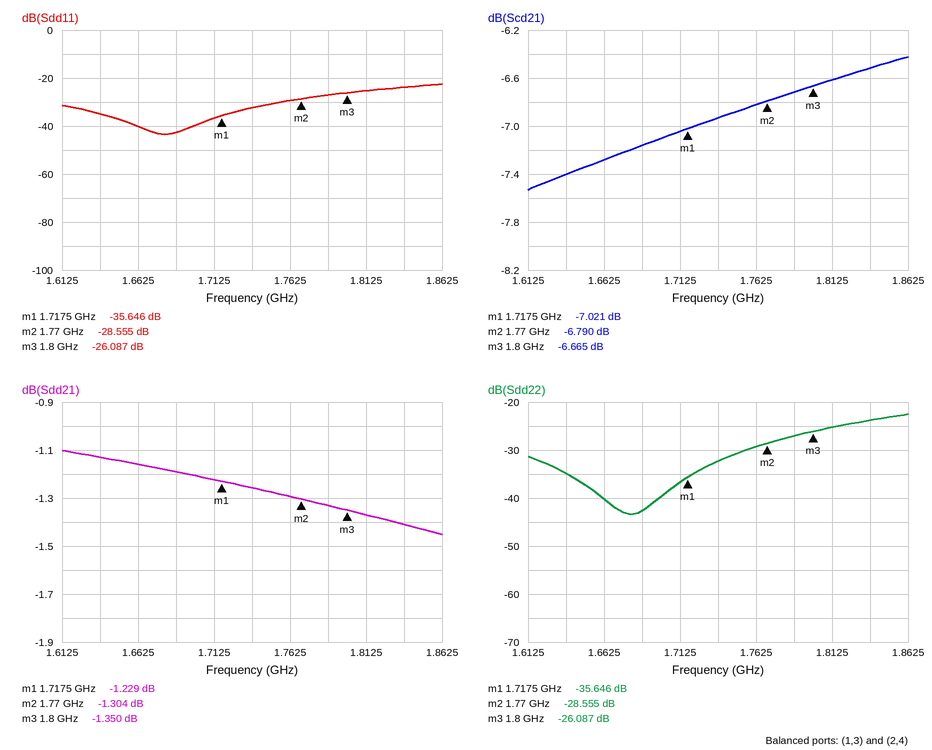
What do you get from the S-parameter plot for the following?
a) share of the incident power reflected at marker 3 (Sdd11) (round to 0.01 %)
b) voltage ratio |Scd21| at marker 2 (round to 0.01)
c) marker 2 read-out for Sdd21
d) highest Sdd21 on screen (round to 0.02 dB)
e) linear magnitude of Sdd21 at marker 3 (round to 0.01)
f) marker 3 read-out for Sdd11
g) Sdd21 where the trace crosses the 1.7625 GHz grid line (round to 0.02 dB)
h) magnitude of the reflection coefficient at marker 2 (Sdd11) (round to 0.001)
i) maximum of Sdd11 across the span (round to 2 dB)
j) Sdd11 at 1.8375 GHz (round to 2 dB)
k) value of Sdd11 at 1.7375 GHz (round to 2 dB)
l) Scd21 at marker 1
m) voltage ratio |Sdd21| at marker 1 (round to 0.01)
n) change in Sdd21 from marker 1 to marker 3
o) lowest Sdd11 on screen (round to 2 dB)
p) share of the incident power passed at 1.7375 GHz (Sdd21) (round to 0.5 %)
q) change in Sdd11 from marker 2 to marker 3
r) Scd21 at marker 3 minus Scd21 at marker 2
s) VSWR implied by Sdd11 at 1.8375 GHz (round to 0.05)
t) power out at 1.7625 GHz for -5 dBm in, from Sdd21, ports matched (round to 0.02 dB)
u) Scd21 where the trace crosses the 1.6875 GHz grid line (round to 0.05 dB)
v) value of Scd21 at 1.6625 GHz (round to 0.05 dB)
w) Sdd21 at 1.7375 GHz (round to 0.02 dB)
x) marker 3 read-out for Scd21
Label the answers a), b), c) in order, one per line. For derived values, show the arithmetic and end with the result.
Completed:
a) 10^(-26.087/10) ≈ 0.25 %
b) 10^(-6.79/20) ≈ 0.46
c) -1.304 dB
d) -1.10 dB
e) 10^(-1.35/20) ≈ 0.86
f) -26.087 dB
g) -1.30 dB
h) 10^(-28.555/20) ≈ 0.037
i) -22 dB
j) -24 dB
k) -32 dB
l) -7.021 dB
m) 10^(-1.229/20) ≈ 0.87
n) -1.35 − (-1.229) = -0.121 dB
o) -44 dB
p) 10^(-1.26/10) ≈ 74.8 %, so 75.0 % to the nearest 0.5 %
q) -26.087 − (-28.555) = 2.468 dB
r) -6.665 − (-6.79) = 0.125 dB
s) |Γ| = 10^(-24/20) = 0.0631; VSWR = (1 + 0.0631)/(1 − 0.0631) ≈ 1.13, so 1.15 to the nearest 0.05
t) -5 dBm + (-1.30 dB) = -6.30 dBm
u) -7.15 dB
v) -7.30 dB
w) -1.26 dB
x) -6.665 dB
